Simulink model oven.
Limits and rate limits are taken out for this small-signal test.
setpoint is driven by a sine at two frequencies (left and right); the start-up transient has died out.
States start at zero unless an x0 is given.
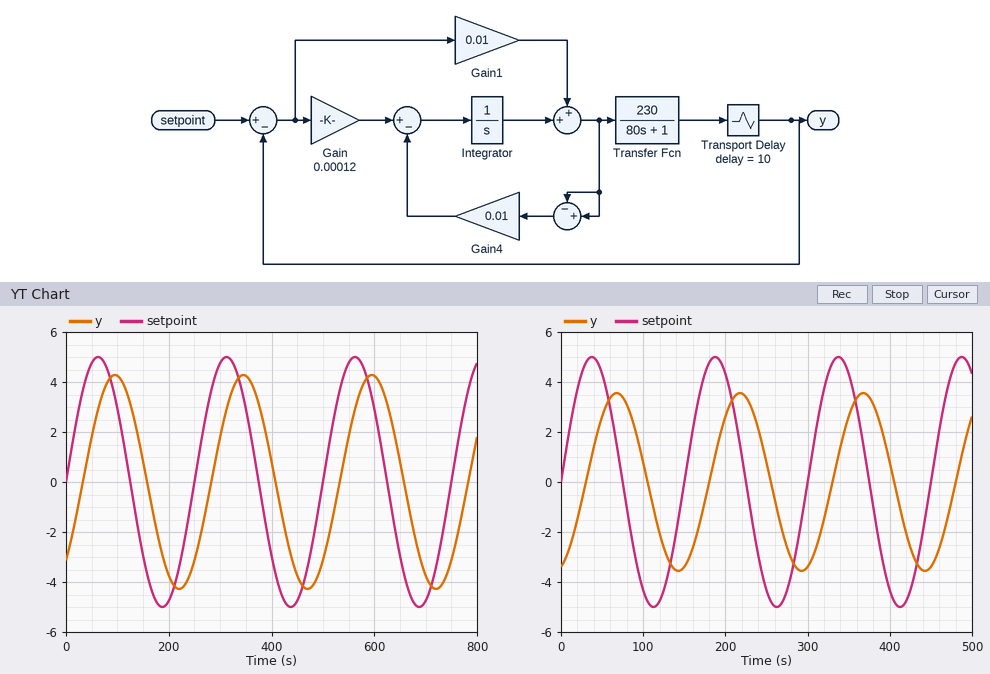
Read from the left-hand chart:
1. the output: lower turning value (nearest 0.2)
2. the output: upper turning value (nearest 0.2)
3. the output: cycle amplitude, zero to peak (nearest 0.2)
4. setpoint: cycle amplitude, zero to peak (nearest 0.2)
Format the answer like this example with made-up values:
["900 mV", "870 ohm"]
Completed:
["-4.2", "4.2", "4.2", "5.0"]
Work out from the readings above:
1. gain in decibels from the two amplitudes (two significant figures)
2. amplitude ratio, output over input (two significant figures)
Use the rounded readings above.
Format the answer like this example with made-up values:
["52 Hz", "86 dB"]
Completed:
["-1.5 dB", "0.84"]
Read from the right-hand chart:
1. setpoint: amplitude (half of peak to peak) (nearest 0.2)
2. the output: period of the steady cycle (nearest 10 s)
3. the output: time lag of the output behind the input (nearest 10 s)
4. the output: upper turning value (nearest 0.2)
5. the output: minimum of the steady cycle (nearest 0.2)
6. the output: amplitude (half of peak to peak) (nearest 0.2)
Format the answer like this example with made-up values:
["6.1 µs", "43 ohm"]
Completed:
["5.0", "150 s", "30 s", "3.6", "-3.6", "3.6"]
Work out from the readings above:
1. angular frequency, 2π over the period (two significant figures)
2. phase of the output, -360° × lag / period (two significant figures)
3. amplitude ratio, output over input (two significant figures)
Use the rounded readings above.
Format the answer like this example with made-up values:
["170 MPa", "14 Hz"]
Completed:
["0.042 rad/s", "-72°", "0.72"]
